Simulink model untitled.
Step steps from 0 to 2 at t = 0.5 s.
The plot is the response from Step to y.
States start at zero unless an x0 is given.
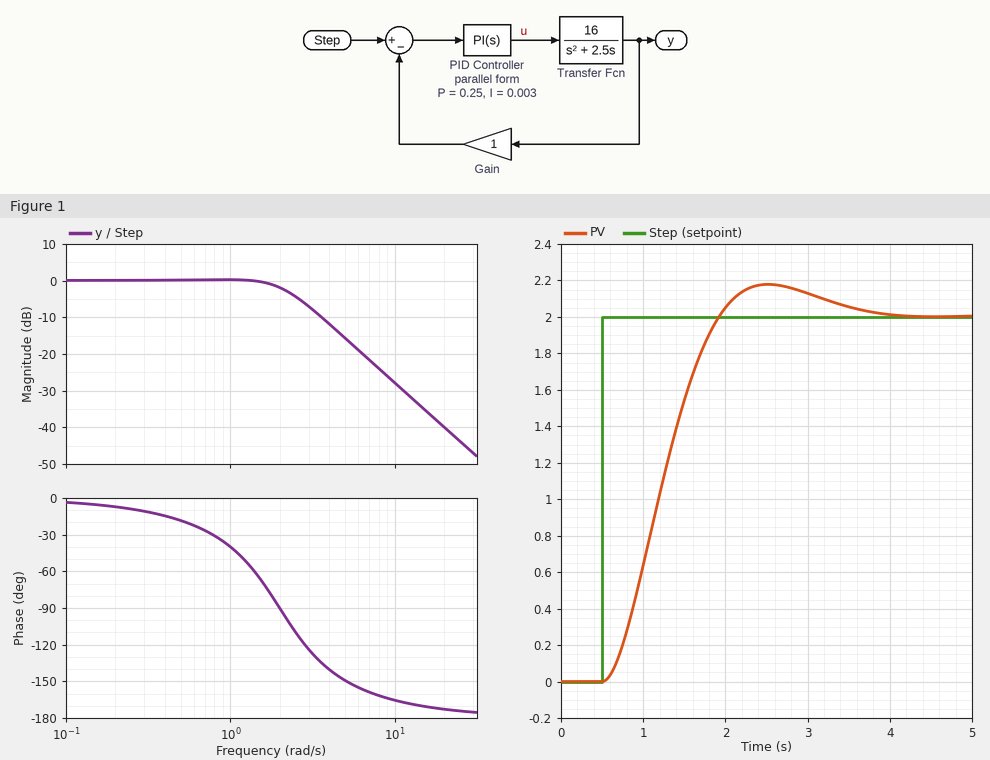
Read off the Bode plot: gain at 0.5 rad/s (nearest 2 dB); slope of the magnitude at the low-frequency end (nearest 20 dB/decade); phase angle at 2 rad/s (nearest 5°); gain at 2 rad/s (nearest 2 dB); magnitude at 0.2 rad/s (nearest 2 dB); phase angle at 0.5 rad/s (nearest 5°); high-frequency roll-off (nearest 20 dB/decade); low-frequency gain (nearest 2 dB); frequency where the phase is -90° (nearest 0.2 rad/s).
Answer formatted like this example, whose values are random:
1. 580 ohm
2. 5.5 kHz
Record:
1. 0 dB
2. 0 dB/decade
3. -90°
4. -2 dB
5. 0 dB
6. -20°
7. -40 dB/decade
8. 0 dB
9. 2.0 rad/s
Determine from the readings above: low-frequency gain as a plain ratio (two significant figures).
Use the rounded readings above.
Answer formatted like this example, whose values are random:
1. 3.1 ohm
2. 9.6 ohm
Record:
1. 1.0
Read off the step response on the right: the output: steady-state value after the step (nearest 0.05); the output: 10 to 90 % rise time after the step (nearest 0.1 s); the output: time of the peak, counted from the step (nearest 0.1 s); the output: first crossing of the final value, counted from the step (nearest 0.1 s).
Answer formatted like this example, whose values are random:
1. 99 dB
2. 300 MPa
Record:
1. 2.00
2. 1.0 s
3. 2.0 s
4. 1.4 s
